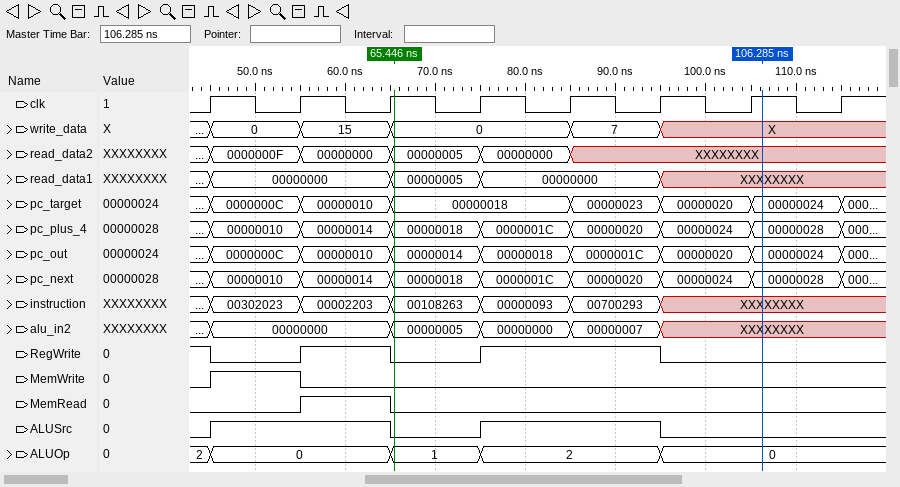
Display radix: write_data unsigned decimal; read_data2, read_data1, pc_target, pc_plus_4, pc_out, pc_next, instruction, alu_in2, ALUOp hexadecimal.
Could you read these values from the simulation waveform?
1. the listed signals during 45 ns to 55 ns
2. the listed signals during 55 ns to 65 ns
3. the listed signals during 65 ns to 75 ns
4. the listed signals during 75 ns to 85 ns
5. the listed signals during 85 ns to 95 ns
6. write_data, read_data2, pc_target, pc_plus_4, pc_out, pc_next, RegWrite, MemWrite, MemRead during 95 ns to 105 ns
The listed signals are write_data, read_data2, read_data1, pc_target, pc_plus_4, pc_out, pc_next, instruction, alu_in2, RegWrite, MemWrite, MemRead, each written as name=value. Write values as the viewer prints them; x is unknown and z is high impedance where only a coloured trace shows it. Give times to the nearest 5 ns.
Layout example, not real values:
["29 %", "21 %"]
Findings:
["write_data=0, read_data2=0000000F, read_data1=00000000, pc_target=0000000C, pc_plus_4=00000010, pc_out=0000000C, pc_next=00000010, instruction=00302023, alu_in2=00000000, RegWrite=0, MemWrite=1, MemRead=0", "write_data=15, read_data2=00000000, read_data1=00000000, pc_target=00000010, pc_plus_4=00000014, pc_out=00000010, pc_next=00000014, instruction=00002203, alu_in2=00000000, RegWrite=1, MemWrite=0, MemRead=1", "write_data=0, read_data2=00000005, read_data1=00000005, pc_target=00000018, pc_plus_4=00000018, pc_out=00000014, pc_next=00000018, instruction=00108263, alu_in2=00000005, RegWrite=0, MemWrite=0, MemRead=0", "write_data=0, read_data2=00000000, read_data1=00000000, pc_target=00000018, pc_plus_4=0000001C, pc_out=00000018, pc_next=0000001C, instruction=00000093, alu_in2=00000000, RegWrite=1, MemWrite=0, MemRead=0", "write_data=7, read_data2=XXXXXXXX, read_data1=00000000, pc_target=00000023, pc_plus_4=00000020, pc_out=0000001C, pc_next=00000020, instruction=00700293, alu_in2=00000007, RegWrite=1, MemWrite=0, MemRead=0", "write_data=X, read_data2=XXXXXXXX, pc_target=00000020, pc_plus_4=00000024, pc_out=00000020, pc_next=00000024, RegWrite=0, MemWrite=0, MemRead=0"]
